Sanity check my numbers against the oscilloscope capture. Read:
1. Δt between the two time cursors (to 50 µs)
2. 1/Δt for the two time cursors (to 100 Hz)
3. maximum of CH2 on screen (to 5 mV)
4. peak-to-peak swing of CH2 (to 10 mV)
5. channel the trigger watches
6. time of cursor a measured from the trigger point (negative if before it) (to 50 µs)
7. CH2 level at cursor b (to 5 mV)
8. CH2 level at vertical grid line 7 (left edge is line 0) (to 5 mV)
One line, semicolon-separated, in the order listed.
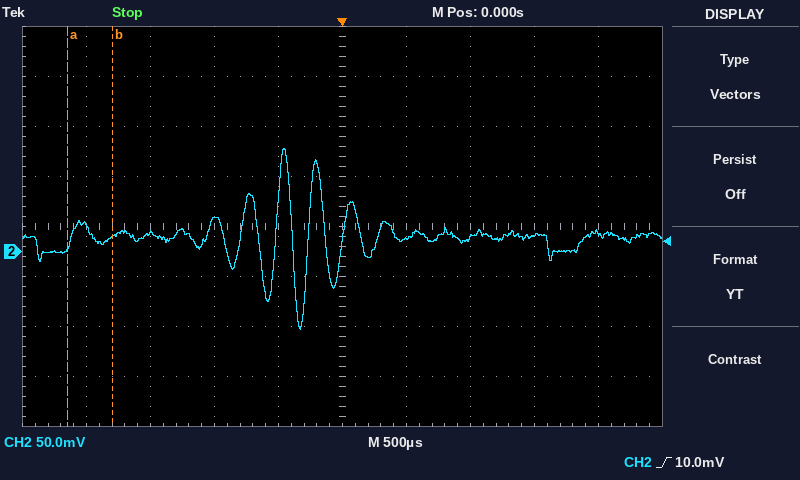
350 µs; 2.9 kHz; 105 mV; 180 mV; CH2; -2.15 ms; 15 mV; 15 mV
